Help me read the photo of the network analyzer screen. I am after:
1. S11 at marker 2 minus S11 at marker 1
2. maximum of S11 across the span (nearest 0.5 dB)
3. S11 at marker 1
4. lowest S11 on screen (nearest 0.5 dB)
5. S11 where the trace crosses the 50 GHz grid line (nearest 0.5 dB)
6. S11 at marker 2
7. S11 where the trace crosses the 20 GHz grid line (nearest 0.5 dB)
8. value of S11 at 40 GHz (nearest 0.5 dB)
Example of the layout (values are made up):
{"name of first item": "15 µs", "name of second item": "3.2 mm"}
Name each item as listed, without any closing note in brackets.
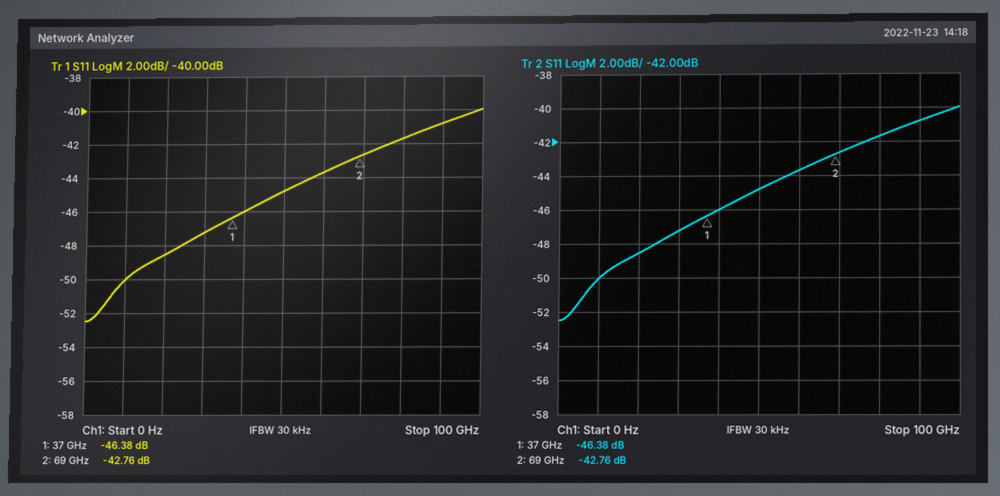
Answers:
{"S11 at marker 2 minus S11 at marker 1": "3.62 dB", "maximum of S11 across the span": "-40.0 dB", "S11 at marker 1": "-46.38 dB", "lowest S11 on screen": "-52.5 dB", "S11 where the trace crosses the 50 GHz grid line": "-45.0 dB", "S11 at marker 2": "-42.76 dB", "S11 where the trace crosses the 20 GHz grid line": "-48.5 dB", "value of S11 at 40 GHz": "-46.0 dB"}
